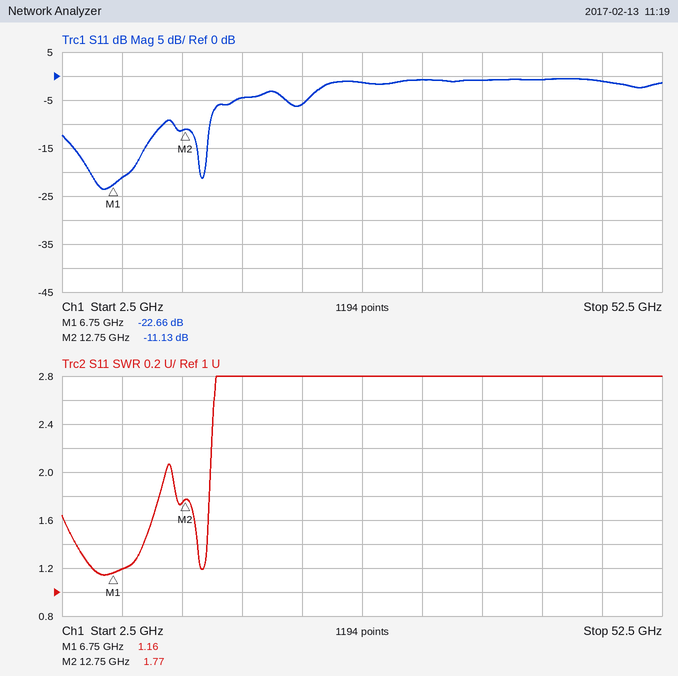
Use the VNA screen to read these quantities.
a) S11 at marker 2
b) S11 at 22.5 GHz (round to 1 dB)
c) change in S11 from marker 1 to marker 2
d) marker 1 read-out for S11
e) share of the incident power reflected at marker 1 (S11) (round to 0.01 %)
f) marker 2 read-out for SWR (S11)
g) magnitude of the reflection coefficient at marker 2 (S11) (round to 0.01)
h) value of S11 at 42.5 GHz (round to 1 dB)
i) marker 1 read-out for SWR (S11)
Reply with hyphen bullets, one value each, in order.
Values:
- -11.13 dB
- -6 dB
- 11.53 dB
- -22.66 dB
- 0.54 %
- 1.77
- 0.28
- -1 dB
- 1.16
